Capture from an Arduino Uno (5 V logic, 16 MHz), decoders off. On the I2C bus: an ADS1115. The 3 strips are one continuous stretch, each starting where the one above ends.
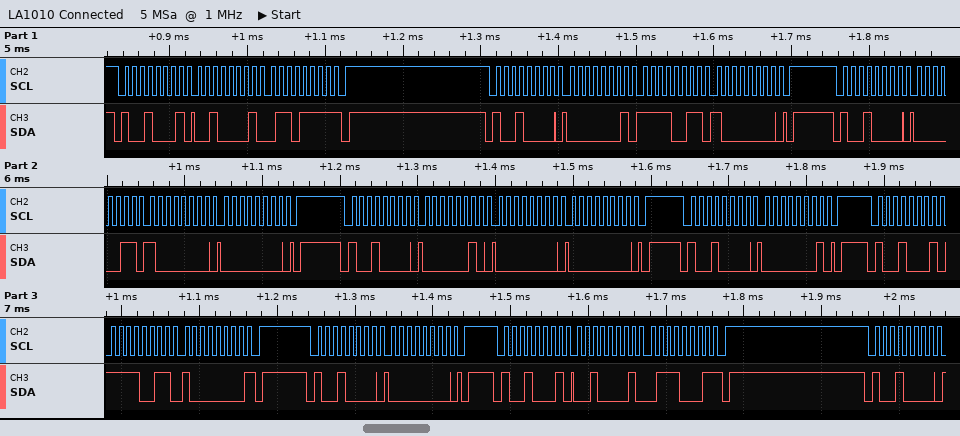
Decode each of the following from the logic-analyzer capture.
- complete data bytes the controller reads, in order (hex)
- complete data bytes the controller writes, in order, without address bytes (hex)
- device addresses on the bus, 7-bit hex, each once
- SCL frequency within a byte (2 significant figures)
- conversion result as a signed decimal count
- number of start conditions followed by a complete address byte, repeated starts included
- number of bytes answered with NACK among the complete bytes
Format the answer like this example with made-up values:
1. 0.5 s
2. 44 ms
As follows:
1. 21 6F F3 80 21 71
2. 01 F3 80 03 80 00 02 00 00 01 00
3. 0x48
4. 100 kHz
5. 8561
6. 9
7. 3
